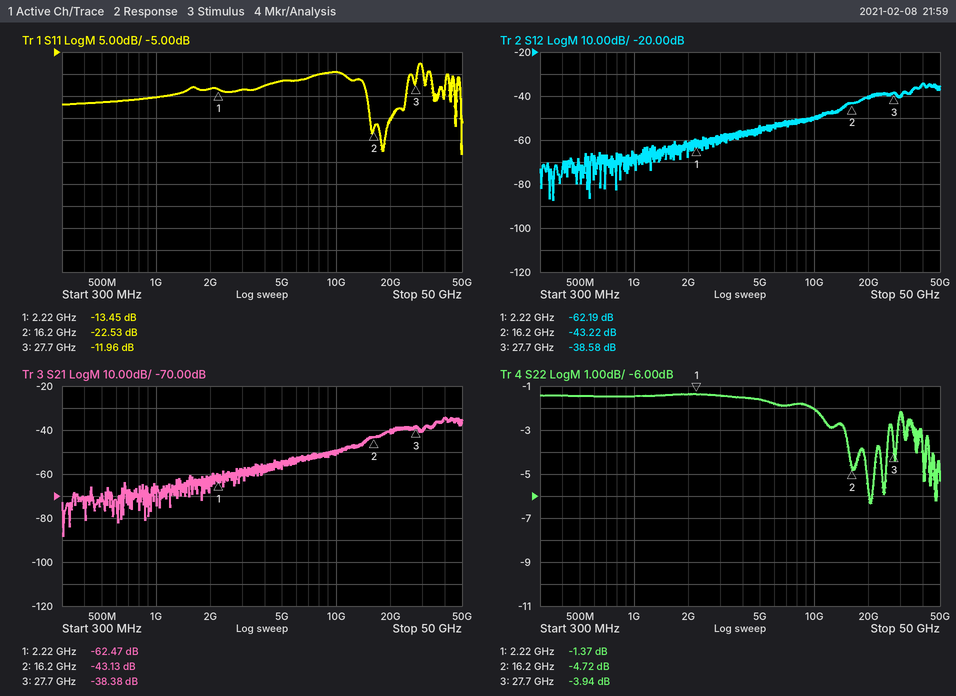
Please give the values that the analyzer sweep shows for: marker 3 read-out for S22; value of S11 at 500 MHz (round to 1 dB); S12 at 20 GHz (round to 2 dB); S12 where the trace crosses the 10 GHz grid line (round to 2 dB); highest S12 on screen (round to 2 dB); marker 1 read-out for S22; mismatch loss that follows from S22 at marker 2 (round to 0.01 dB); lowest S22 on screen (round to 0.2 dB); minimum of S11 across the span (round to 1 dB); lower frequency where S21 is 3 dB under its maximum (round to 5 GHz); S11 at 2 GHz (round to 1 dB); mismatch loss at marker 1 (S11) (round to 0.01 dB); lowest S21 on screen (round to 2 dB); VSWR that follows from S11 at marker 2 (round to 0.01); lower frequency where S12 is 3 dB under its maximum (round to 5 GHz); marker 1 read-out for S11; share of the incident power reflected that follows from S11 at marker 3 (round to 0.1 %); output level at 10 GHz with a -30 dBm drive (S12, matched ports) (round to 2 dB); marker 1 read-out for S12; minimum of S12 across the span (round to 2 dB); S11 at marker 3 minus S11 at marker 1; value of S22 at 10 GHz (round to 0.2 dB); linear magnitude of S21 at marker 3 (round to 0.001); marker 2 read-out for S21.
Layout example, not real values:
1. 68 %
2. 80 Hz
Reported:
1. -3.94 dB
2. -16 dB
3. -40 dB
4. -50 dB
5. -34 dB
6. -1.37 dB
7. 1.79 dB
8. -6.4 dB
9. -28 dB
10. 35 GHz
11. -13 dB
12. 0.20 dB
13. -88 dB
14. 1.16
15. 35 GHz
16. -13.45 dB
17. 6.4 %
18. -80 dBm
19. -62.19 dB
20. -88 dB
21. 1.49 dB
22. -2.0 dB
23. 0.012
24. -43.13 dB
